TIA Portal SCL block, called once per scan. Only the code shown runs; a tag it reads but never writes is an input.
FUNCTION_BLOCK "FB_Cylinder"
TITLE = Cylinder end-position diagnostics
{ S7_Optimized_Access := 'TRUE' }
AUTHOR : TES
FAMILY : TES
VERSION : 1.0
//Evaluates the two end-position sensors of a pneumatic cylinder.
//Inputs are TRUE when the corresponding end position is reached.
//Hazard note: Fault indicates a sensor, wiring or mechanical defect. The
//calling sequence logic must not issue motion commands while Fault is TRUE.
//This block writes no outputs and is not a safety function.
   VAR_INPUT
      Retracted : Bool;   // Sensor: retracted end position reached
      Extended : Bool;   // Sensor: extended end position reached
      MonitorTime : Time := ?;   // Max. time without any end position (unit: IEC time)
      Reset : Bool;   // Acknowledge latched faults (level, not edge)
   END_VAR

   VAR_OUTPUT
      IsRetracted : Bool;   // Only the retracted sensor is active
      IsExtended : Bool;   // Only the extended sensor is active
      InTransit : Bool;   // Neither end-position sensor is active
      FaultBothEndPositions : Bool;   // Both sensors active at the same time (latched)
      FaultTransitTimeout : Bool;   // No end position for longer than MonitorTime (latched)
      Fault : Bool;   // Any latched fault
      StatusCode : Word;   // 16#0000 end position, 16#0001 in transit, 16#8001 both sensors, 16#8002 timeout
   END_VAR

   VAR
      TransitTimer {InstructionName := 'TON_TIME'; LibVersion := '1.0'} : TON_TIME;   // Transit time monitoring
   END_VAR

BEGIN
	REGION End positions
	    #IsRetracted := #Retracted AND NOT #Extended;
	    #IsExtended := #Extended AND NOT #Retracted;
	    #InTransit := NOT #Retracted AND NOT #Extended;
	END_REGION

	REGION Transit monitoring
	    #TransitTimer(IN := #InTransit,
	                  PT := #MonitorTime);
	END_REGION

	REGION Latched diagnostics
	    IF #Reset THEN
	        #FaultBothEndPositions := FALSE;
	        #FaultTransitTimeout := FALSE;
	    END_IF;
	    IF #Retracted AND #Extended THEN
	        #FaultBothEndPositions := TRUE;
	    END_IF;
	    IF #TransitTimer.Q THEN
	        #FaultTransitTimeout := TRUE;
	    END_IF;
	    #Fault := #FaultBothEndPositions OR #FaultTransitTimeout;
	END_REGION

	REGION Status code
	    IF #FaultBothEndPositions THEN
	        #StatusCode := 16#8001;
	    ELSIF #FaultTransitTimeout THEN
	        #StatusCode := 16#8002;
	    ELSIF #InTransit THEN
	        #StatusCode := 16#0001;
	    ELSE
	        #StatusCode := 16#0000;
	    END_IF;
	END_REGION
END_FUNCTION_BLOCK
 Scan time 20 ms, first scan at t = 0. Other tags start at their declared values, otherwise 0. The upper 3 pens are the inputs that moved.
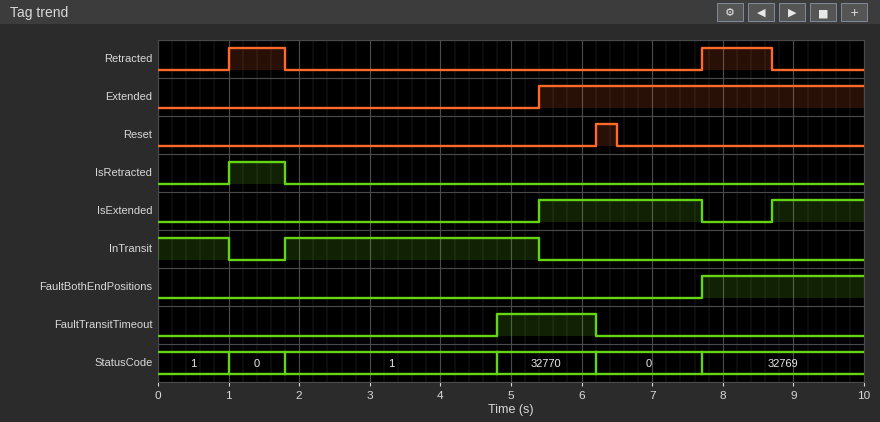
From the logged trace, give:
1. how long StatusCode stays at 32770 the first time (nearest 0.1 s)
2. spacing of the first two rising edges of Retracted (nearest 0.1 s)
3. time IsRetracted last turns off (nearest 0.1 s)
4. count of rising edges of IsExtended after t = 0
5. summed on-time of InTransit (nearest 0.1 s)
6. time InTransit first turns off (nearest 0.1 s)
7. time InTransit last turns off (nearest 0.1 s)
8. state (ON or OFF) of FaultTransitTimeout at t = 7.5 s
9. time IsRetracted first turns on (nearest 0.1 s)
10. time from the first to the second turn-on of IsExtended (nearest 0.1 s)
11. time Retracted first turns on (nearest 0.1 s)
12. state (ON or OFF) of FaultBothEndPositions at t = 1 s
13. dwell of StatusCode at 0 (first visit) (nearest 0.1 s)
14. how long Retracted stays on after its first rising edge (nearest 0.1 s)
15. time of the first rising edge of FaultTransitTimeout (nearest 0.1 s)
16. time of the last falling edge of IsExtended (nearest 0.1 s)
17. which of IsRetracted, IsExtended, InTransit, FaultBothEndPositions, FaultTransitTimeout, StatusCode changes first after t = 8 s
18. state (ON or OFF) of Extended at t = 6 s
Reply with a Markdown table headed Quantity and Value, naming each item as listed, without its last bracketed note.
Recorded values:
| Quantity | Value |
|---|---|
| how long StatusCode stays at 32770 the first time | 1.4 s |
| spacing of the first two rising edges of Retracted | 6.7 s |
| time IsRetracted last turns off | 1.8 s |
| count of rising edges of IsExtended after t = 0 | 2 |
| summed on-time of InTransit | 4.6 s |
| time InTransit first turns off | 1.0 s |
| time InTransit last turns off | 5.4 s |
| state (ON or OFF) of FaultTransitTimeout at t = 7.5 s | OFF |
| time IsRetracted first turns on | 1.0 s |
| time from the first to the second turn-on of IsExtended | 3.3 s |
| time Retracted first turns on | 1.0 s |
| state (ON or OFF) of FaultBothEndPositions at t = 1 s | OFF |
| dwell of StatusCode at 0 (first visit) | 0.8 s |
| how long Retracted stays on after its first rising edge | 0.8 s |
| time of the first rising edge of FaultTransitTimeout | 4.8 s |
| time of the last falling edge of IsExtended | 7.7 s |
| which of IsRetracted, IsExtended, InTransit, FaultBothEndPositions, FaultTransitTimeout, StatusCode changes first after t = 8 s | IsExtended |
| state (ON or OFF) of Extended at t = 6 s | ON |
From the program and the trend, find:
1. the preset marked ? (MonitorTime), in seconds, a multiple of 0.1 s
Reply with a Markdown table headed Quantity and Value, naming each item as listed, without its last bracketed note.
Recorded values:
| Quantity | Value |
|---|---|
| the preset marked ? (MonitorTime), in seconds, a multiple of 0.1 s | 3.0 s |
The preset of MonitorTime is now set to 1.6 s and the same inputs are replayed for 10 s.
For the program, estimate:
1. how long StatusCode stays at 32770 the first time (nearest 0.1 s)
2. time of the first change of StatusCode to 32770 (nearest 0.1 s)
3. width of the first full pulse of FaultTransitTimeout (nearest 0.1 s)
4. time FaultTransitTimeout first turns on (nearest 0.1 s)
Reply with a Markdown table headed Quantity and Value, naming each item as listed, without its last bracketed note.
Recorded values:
| Quantity | Value |
|---|---|
| how long StatusCode stays at 32770 the first time | 2.8 s |
| time of the first change of StatusCode to 32770 | 3.4 s |
| width of the first full pulse of FaultTransitTimeout | 2.8 s |
| time FaultTransitTimeout first turns on | 3.4 s |
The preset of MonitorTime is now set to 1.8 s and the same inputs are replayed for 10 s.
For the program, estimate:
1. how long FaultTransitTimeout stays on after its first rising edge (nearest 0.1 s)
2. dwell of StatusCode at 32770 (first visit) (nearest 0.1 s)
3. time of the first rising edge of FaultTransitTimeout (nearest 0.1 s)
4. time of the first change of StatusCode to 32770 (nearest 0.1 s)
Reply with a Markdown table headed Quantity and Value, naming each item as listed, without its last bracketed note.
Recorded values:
| Quantity | Value |
|---|---|
| how long FaultTransitTimeout stays on after its first rising edge | 2.6 s |
| dwell of StatusCode at 32770 (first visit) | 2.6 s |
| time of the first rising edge of FaultTransitTimeout | 3.6 s |
| time of the first change of StatusCode to 32770 | 3.6 s |
